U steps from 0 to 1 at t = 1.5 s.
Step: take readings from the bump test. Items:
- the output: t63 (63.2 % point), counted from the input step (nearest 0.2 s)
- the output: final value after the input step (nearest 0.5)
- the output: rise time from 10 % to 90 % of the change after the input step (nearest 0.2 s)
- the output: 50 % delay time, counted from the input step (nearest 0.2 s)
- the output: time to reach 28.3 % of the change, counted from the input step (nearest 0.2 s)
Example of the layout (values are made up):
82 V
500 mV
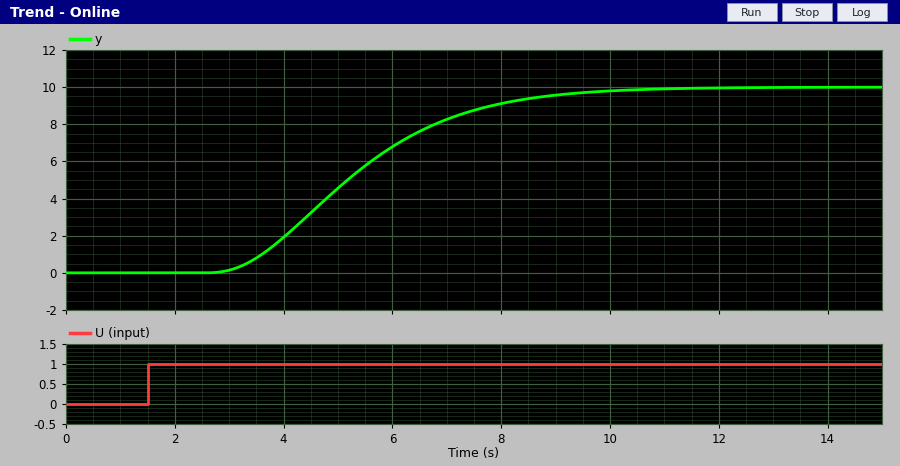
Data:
4.2 s
10.0
4.2 s
3.6 s
2.8 s
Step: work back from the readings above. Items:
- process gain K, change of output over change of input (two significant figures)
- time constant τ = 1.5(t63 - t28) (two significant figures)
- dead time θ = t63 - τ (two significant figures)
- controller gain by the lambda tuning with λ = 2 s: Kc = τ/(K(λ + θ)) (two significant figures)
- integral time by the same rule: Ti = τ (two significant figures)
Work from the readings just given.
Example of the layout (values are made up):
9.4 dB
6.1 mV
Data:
10
2.1 s
2.1 s
0.051
2.1 s
